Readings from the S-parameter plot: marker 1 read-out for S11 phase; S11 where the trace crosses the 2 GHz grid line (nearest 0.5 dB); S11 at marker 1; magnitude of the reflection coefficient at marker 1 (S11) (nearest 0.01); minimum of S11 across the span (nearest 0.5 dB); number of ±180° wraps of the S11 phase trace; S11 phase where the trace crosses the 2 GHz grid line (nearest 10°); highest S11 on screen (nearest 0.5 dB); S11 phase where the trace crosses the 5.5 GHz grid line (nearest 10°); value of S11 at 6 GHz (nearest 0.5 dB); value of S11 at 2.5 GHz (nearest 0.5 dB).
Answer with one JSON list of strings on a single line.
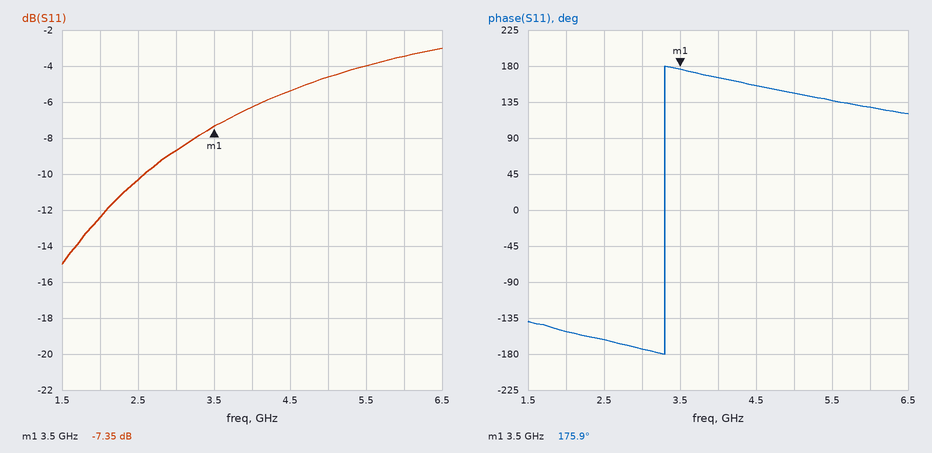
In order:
["175.9°", "-12.5 dB", "-7.35 dB", "0.43", "-15.0 dB", "1", "-150°", "-3.0 dB", "140°", "-3.5 dB", "-10.5 dB"]
